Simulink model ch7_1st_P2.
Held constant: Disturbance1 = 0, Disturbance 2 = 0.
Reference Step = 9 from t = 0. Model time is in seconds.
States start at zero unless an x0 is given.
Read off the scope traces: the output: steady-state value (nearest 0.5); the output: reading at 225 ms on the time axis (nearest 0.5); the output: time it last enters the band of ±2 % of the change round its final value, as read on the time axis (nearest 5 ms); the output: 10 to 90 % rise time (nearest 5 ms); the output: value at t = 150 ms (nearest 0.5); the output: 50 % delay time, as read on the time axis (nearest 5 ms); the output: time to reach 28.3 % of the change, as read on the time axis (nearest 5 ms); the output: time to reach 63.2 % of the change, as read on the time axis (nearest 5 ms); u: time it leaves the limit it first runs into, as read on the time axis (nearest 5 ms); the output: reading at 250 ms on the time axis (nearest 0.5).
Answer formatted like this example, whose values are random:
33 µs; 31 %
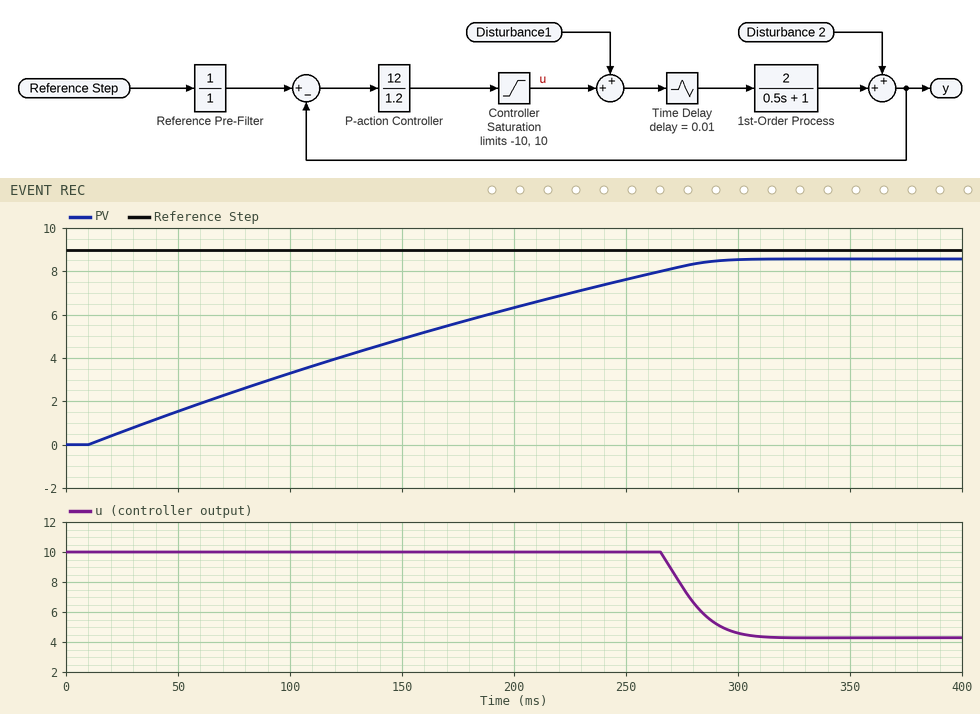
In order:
8.5; 7.0; 285 ms; 220 ms; 5.0; 130 ms; 75 ms; 170 ms; 265 ms; 7.5
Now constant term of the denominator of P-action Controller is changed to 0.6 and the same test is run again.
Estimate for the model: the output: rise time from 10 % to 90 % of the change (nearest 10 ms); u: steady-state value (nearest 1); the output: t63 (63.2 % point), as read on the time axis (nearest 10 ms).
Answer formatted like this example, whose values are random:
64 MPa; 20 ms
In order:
230 ms; 4; 170 ms
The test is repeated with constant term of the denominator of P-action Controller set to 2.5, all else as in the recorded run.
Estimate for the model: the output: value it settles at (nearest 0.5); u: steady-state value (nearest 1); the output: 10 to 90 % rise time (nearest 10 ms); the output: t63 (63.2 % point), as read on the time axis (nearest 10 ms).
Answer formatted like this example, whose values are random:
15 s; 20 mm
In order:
8.0; 4; 210 ms; 160 ms
